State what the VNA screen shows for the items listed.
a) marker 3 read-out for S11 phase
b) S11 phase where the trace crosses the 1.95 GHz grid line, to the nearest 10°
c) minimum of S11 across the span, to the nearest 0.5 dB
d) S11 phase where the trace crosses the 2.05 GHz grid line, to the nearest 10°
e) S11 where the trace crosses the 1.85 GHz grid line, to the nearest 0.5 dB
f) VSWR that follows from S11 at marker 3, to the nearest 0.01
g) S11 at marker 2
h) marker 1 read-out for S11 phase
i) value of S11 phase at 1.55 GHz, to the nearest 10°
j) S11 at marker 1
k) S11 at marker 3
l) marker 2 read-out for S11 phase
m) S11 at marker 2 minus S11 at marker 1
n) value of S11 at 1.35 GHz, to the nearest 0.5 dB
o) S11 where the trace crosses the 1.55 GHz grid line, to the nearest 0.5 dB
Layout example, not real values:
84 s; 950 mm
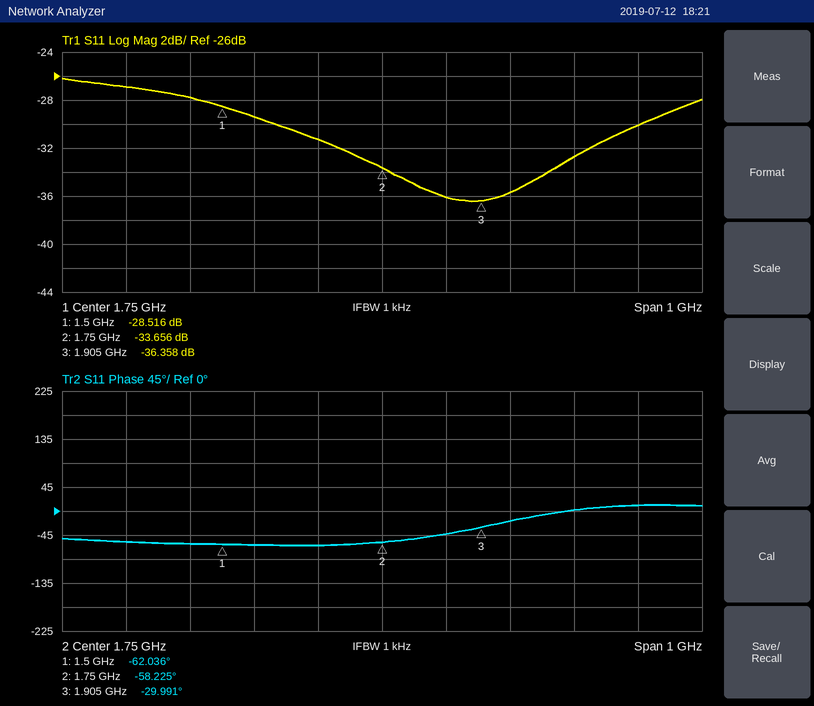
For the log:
-29.991°; -20°; -36.5 dB; 0°; -36.0 dB; 1.03; -33.656 dB; -62.036°; -60°; -28.516 dB; -36.358 dB; -58.225°; -5.140 dB; -27.0 dB; -29.5 dB
